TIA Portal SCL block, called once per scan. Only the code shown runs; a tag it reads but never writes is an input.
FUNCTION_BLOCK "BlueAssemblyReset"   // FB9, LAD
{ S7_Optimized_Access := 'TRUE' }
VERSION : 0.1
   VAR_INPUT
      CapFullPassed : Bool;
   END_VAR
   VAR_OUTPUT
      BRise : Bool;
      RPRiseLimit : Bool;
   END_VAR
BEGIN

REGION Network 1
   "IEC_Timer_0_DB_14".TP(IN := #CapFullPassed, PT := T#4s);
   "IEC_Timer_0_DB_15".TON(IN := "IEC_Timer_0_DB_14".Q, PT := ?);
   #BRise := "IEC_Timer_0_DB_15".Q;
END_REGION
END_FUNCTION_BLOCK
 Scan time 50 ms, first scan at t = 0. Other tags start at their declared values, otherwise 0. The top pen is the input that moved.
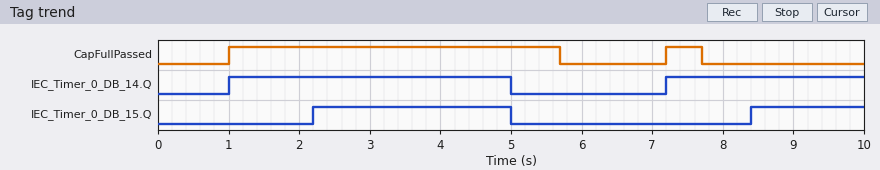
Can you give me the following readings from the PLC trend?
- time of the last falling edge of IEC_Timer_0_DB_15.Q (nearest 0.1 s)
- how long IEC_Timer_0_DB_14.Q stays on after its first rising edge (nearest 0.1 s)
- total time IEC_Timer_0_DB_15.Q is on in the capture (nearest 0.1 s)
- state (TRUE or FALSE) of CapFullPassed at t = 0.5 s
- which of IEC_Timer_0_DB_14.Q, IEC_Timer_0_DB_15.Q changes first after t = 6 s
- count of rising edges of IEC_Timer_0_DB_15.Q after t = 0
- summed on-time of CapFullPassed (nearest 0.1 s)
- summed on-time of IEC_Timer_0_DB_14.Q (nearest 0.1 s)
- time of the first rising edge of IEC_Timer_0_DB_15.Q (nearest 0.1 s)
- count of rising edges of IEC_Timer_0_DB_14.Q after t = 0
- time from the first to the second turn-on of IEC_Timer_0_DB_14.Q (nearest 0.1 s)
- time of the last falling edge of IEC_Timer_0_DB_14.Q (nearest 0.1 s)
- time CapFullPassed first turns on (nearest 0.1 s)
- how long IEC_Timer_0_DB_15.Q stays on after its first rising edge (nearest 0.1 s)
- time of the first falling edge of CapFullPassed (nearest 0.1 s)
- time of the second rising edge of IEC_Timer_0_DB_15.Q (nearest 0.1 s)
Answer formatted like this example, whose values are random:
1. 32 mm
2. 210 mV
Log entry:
1. 5.0 s
2. 4.0 s
3. 4.4 s
4. FALSE
5. IEC_Timer_0_DB_14.Q
6. 2
7. 5.2 s
8. 6.8 s
9. 2.2 s
10. 2
11. 6.2 s
12. 5.0 s
13. 1.0 s
14. 2.8 s
15. 5.7 s
16. 8.4 s
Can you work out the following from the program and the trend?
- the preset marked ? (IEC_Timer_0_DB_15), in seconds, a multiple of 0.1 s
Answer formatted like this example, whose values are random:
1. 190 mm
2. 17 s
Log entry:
1. 1.2 s
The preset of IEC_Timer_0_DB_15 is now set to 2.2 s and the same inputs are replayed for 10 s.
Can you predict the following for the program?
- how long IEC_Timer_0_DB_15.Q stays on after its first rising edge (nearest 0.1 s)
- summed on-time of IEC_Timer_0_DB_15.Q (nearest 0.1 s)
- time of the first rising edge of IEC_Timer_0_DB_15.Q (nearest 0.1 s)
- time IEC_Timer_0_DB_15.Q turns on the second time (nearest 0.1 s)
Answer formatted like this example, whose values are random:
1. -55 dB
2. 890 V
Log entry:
1. 1.8 s
2. 2.4 s
3. 3.2 s
4. 9.4 s
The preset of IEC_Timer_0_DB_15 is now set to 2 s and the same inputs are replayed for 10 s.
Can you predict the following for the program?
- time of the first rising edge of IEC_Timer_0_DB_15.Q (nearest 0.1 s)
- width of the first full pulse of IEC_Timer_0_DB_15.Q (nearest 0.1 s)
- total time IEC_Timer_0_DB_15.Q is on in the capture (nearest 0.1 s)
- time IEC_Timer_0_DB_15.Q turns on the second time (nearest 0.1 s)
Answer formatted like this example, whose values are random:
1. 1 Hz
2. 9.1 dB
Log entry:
1. 3.0 s
2. 2.0 s
3. 2.8 s
4. 9.2 s
